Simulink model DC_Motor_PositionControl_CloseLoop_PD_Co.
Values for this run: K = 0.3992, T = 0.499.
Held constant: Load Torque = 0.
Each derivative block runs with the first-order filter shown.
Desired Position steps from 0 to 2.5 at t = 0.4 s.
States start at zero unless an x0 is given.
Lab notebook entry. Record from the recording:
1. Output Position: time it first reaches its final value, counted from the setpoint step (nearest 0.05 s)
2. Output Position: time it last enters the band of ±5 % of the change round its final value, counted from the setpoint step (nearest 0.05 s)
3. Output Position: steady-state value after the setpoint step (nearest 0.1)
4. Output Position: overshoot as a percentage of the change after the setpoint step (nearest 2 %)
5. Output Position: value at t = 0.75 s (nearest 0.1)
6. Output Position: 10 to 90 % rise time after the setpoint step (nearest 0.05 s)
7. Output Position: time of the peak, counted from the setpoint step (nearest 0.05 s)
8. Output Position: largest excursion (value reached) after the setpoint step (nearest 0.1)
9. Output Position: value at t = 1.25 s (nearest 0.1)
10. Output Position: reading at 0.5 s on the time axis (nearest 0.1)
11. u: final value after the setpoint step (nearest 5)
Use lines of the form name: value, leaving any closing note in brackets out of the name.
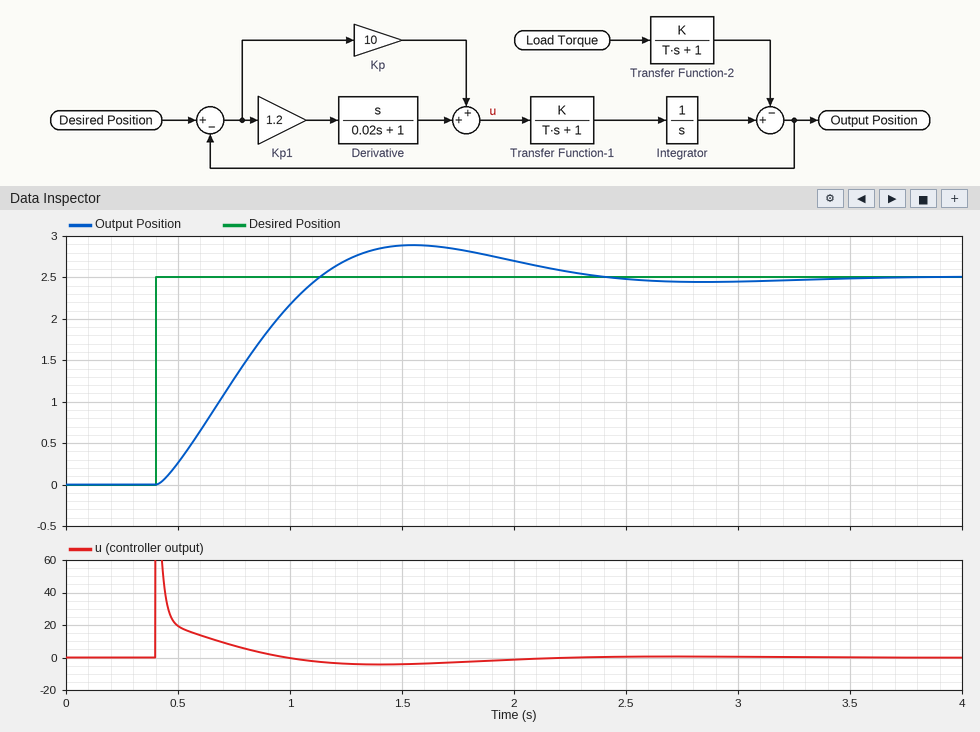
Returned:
Output Position: time it first reaches its final value, counted from the setpoint step: 0.75 s
Output Position: time it last enters the band of ±5 % of the change round its final value, counted from the setpoint step: 1.75 s
Output Position: steady-state value after the setpoint step: 2.5
Output Position: overshoot as a percentage of the change after the setpoint step: 16 %
Output Position: value at t = 0.75 s: 1.3
Output Position: 10 to 90 % rise time after the setpoint step: 0.55 s
Output Position: time of the peak, counted from the setpoint step: 1.15 s
Output Position: largest excursion (value reached) after the setpoint step: 2.9
Output Position: value at t = 1.25 s: 2.7
Output Position: reading at 0.5 s on the time axis: 0.3
u: final value after the setpoint step: 0
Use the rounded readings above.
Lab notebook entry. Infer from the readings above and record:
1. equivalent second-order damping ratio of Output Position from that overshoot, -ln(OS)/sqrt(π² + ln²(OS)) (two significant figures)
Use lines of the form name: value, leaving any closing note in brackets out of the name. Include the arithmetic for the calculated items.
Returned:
equivalent second-order damping ratio of Output Position from that overshoot, -ln(OS)/sqrt(π² + ln²(OS)): ln(0.16) = -1.833; 1.833 / sqrt(9.870 + 3.358) = 0.50
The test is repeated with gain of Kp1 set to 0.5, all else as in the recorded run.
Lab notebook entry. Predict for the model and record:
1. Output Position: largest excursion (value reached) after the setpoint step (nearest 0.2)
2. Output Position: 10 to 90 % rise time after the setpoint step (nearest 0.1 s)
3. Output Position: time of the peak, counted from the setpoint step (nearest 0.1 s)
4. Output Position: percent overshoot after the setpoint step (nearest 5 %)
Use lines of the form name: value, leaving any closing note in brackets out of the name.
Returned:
Output Position: largest excursion (value reached) after the setpoint step: 3.0
Output Position: 10 to 90 % rise time after the setpoint step: 0.5 s
Output Position: time of the peak, counted from the setpoint step: 1.2 s
Output Position: percent overshoot after the setpoint step: 25 %
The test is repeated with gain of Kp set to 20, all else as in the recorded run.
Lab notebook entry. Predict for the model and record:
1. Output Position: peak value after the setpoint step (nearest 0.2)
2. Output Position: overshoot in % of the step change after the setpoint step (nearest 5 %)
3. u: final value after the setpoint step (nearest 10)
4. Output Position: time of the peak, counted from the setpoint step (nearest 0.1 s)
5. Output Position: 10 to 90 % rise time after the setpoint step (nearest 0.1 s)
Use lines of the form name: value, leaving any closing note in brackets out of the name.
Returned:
Output Position: peak value after the setpoint step: 3.2
Output Position: overshoot in % of the step change after the setpoint step: 30 %
u: final value after the setpoint step: 0
Output Position: time of the peak, counted from the setpoint step: 0.8 s
Output Position: 10 to 90 % rise time after the setpoint step: 0.3 s
